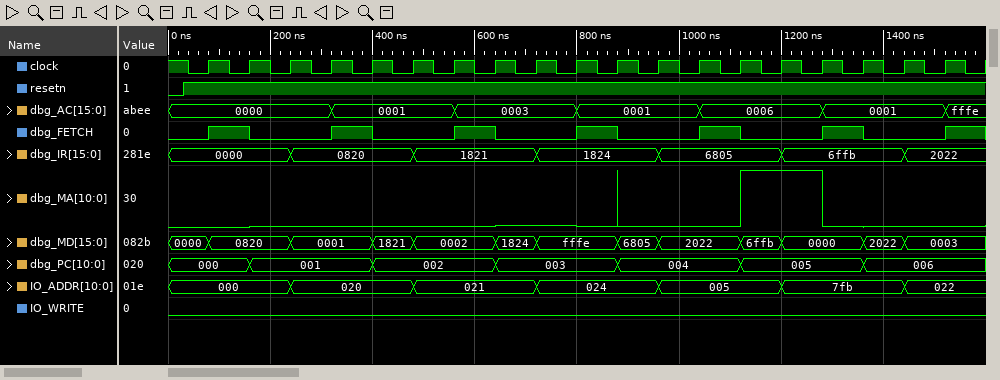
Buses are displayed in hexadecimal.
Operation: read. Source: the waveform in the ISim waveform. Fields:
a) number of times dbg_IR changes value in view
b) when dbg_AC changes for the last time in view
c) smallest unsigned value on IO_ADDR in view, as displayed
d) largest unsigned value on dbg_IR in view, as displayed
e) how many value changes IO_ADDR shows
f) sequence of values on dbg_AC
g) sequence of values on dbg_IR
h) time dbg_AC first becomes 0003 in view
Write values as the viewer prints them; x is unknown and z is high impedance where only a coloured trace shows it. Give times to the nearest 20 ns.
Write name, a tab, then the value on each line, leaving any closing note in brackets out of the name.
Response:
number of times dbg_IR changes value in view	6
when dbg_AC changes for the last time in view	1520 ns
smallest unsigned value on IO_ADDR in view, as displayed	000
largest unsigned value on dbg_IR in view, as displayed	6ffb
how many value changes IO_ADDR shows	6
sequence of values on dbg_AC	0000, 0001, 0003, 0001, 0006, 0001, fffe
sequence of values on dbg_IR	0000, 0820, 1821, 1824, 6805, 6ffb, 2022
time dbg_AC first becomes 0003 in view	560 ns
